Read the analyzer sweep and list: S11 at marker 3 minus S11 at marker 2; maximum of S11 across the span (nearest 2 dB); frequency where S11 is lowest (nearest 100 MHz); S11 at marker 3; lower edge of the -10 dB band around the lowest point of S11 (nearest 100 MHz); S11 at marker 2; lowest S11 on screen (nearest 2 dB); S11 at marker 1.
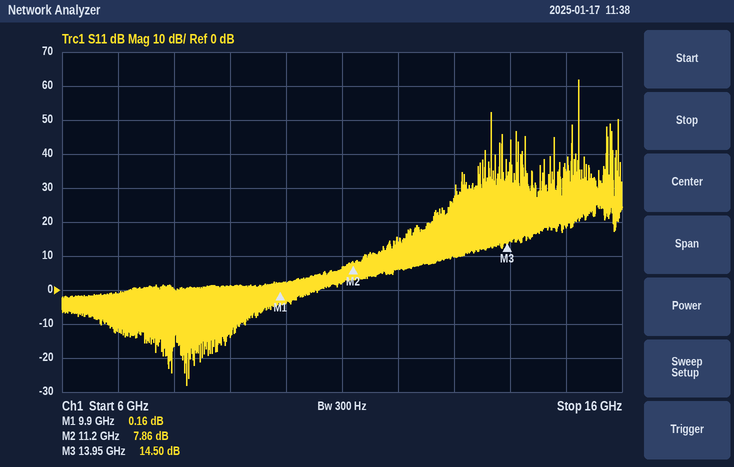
6.64 dB
62 dB
8.2 GHz
14.50 dB
8.2 GHz
7.86 dB
-28 dB
0.16 dB
